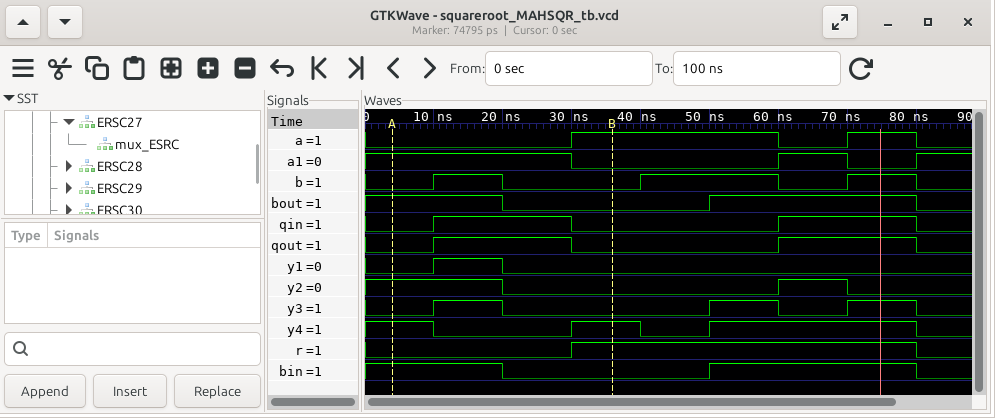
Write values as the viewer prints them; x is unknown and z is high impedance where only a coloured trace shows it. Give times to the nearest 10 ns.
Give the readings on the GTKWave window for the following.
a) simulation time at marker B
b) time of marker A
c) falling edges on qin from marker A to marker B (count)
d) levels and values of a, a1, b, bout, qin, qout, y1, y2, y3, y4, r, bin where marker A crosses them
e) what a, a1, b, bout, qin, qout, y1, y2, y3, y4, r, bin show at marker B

40 ns
0 ns
1
a=0, a1=1, b=0, bout=1, qin=0, qout=0, y1=0, y2=1, y3=0, y4=1, r=0, bin=1
a=1, a1=0, b=0, bout=0, qin=0, qout=0, y1=0, y2=0, y3=0, y4=1, r=1, bin=0
